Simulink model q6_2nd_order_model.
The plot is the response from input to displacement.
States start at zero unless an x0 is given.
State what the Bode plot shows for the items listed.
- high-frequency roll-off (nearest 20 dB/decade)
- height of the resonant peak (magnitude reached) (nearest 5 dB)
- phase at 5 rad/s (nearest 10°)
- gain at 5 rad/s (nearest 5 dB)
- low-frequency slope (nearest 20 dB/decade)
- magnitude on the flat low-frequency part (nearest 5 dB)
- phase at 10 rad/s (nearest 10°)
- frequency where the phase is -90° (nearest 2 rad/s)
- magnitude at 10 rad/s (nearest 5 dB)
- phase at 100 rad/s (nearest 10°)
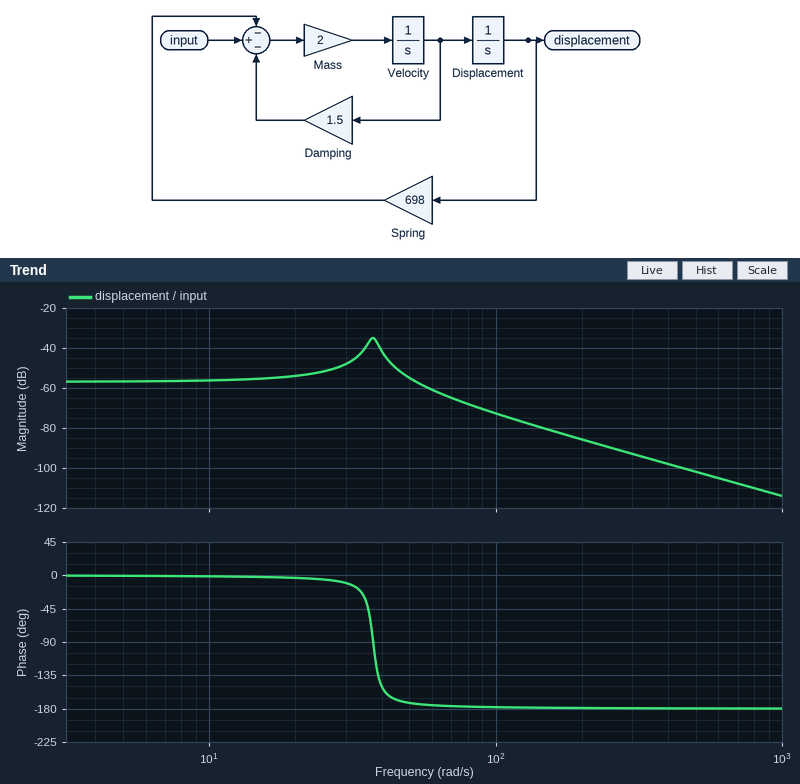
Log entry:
-40 dB/decade
-35 dB
0°
-55 dB
0 dB/decade
-55 dB
0°
38 rad/s
-55 dB
-180°
